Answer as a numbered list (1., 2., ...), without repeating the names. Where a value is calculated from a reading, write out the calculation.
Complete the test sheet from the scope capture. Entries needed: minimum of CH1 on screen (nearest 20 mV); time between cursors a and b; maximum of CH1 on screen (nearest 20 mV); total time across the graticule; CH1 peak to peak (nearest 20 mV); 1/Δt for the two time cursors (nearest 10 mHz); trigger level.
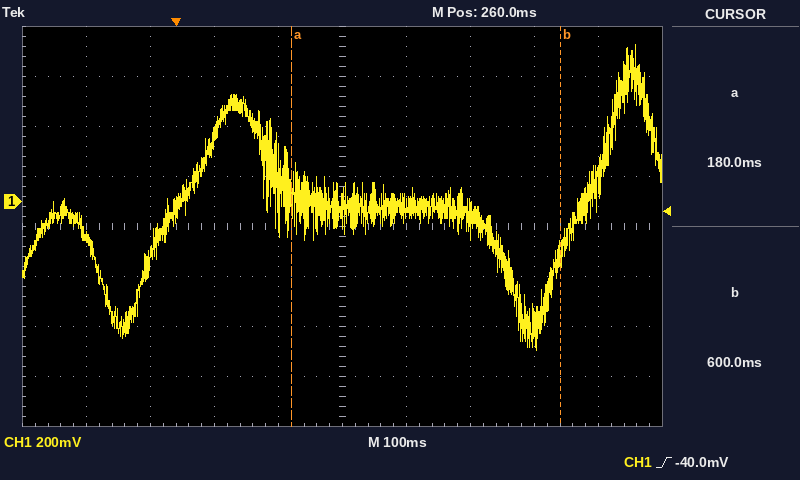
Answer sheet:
1. -600 mV
2. 600 ms − (180 ms) = 420 ms
3. 620 mV
4. 1 s
5. 620 mV − (-600 mV) = 1.22 V
6. 1 / 420 ms ≈ 2.38 Hz
7. -40.0 mV
